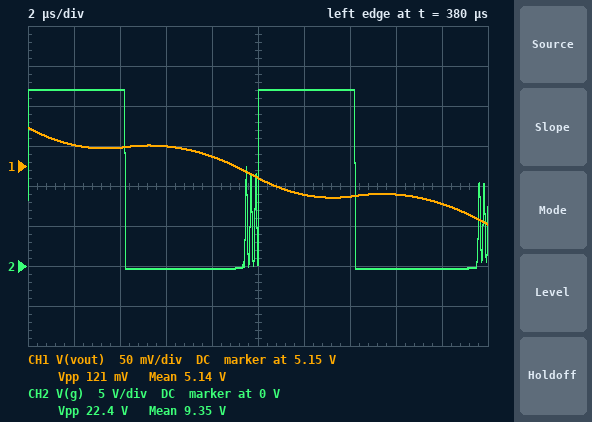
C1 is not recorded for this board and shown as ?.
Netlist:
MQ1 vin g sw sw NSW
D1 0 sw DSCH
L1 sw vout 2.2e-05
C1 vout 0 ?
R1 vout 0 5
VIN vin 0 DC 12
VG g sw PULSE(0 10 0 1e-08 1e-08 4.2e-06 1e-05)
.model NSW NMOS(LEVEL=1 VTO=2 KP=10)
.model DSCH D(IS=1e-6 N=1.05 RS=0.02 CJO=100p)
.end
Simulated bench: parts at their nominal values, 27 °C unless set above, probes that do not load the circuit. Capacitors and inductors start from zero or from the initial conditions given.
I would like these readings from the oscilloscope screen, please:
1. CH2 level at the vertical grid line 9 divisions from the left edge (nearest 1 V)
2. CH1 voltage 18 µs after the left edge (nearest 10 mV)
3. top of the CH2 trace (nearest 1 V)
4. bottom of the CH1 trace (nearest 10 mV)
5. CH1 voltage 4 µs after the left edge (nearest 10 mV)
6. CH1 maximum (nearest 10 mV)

0 V
5.10 V
22 V
5.08 V
5.17 V
5.20 V
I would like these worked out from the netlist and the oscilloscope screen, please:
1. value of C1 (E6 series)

68 µF
